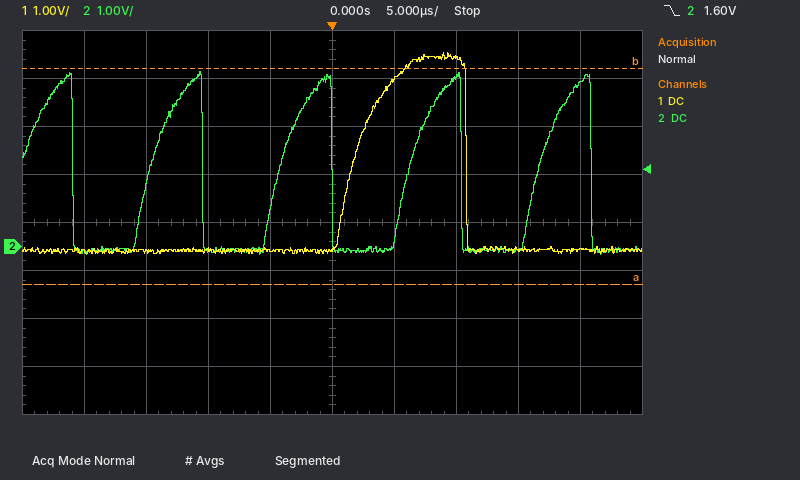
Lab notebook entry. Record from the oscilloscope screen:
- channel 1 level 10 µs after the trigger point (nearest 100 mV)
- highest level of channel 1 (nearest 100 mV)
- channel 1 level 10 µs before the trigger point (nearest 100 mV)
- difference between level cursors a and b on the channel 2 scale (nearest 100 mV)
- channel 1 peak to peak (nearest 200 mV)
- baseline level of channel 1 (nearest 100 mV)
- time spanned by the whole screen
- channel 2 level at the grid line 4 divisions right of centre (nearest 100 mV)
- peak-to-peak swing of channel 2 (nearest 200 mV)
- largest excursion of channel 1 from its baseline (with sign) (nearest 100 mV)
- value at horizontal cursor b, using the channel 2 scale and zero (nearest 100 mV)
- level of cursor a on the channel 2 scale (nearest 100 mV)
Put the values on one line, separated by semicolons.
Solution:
3.9 V; 4.0 V; -100 mV; 4.5 V; 4.2 V; -100 mV; 50 µs; 3.4 V; 3.8 V; +4.1 V; 3.7 V; -800 mV
